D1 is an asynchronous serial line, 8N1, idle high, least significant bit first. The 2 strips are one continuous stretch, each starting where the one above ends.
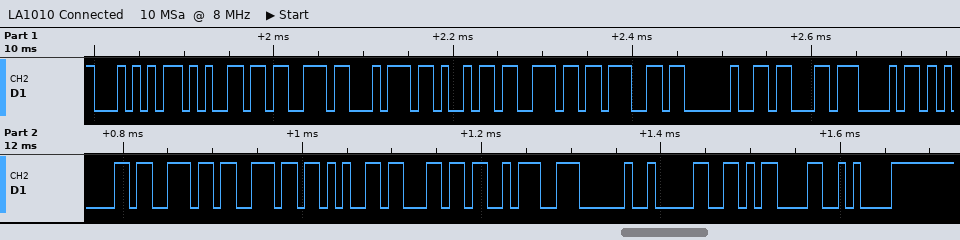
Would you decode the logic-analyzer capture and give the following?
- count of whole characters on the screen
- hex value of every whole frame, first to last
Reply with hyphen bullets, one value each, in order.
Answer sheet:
- 20
- 54 65 73 74 69 6E 67 20 63 68 61 6E 6E 65 6C 3A 20 30 0D 0A
